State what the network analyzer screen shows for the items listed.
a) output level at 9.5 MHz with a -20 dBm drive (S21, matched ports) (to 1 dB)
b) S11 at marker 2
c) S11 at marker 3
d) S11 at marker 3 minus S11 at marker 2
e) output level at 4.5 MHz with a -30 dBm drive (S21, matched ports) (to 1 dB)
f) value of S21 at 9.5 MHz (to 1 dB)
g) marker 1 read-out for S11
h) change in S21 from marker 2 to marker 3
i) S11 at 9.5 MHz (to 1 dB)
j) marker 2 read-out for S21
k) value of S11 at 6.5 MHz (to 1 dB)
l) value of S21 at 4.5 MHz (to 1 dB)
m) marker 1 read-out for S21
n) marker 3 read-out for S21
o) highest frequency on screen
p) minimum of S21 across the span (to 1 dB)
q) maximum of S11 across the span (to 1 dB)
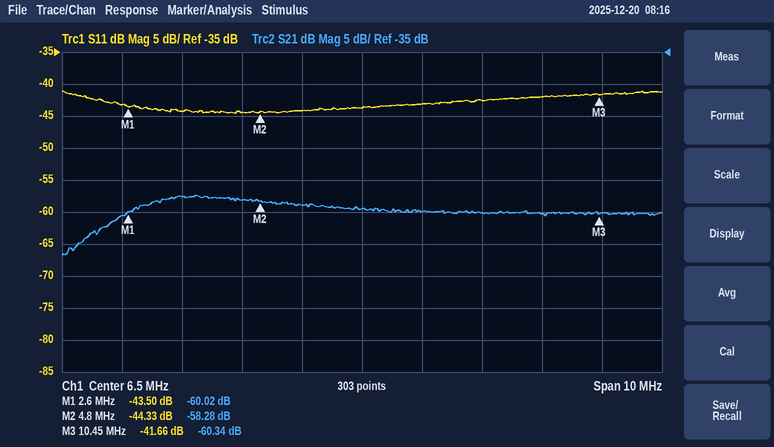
-80 dBm
-44.33 dB
-41.66 dB
2.67 dB
-88 dBm
-60 dB
-43.50 dB
-2.06 dB
-42 dB
-58.28 dB
-44 dB
-58 dB
-60.02 dB
-60.34 dB
11.5 MHz
-67 dB
-41 dB
